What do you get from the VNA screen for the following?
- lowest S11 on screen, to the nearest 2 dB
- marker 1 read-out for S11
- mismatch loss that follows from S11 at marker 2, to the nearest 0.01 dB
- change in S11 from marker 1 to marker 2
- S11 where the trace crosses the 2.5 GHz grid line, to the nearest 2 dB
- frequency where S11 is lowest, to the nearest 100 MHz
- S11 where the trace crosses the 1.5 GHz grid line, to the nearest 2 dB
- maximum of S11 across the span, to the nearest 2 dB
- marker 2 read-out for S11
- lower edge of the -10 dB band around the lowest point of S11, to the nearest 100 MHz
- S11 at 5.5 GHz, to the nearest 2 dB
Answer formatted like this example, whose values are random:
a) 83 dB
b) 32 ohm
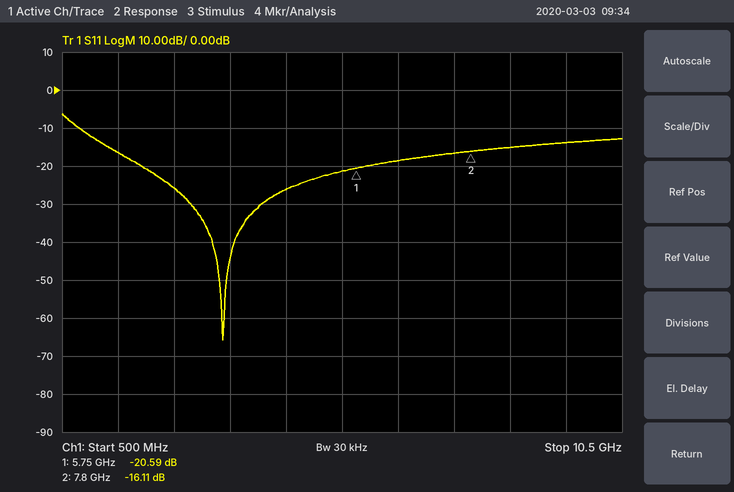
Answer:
a) -66 dB
b) -20.59 dB
c) 0.11 dB
d) 4.48 dB
e) -26 dB
f) 3.4 GHz
g) -16 dB
h) -6 dB
i) -16.11 dB
j) 800 MHz
k) -22 dB
